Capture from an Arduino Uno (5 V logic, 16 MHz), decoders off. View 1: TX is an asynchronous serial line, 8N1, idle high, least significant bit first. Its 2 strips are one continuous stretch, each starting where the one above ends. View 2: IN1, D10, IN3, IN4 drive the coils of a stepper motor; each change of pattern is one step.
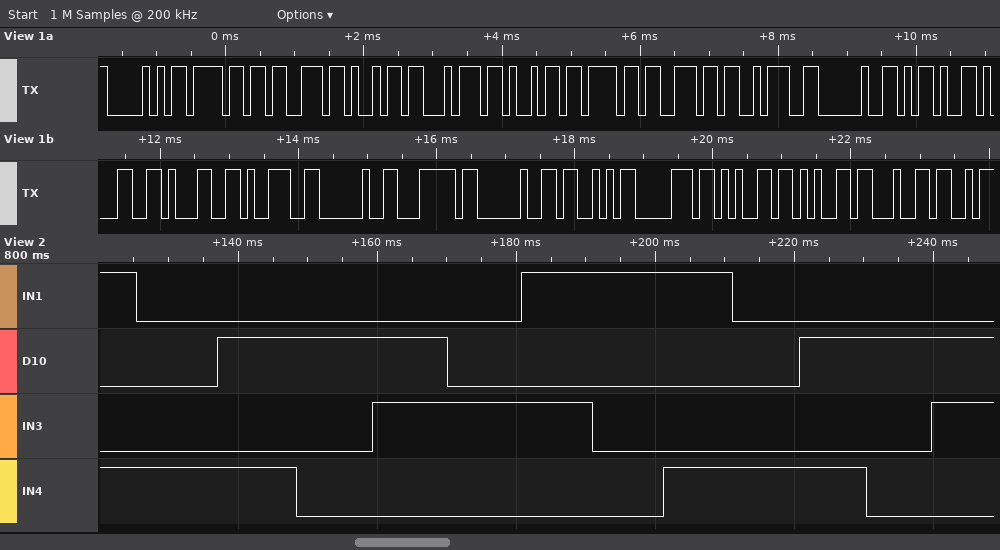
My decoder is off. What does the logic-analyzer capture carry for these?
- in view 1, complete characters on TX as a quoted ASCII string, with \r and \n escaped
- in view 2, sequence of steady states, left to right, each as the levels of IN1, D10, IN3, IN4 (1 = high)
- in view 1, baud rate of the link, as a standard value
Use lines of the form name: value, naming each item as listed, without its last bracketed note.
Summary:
in view 1, complete characters on TX as a quoted ASCII string, with \r and \n escaped: "Position: -119 | Speed"
in view 2, sequence of steady states, left to right, each as the levels of IN1, D10, IN3, IN4: 1001 0001 0101 0100 0110 0010 1010 1000 1001 0001 0101 0100 0110
in view 1, baud rate of the link, as a standard value: 9600 baud
